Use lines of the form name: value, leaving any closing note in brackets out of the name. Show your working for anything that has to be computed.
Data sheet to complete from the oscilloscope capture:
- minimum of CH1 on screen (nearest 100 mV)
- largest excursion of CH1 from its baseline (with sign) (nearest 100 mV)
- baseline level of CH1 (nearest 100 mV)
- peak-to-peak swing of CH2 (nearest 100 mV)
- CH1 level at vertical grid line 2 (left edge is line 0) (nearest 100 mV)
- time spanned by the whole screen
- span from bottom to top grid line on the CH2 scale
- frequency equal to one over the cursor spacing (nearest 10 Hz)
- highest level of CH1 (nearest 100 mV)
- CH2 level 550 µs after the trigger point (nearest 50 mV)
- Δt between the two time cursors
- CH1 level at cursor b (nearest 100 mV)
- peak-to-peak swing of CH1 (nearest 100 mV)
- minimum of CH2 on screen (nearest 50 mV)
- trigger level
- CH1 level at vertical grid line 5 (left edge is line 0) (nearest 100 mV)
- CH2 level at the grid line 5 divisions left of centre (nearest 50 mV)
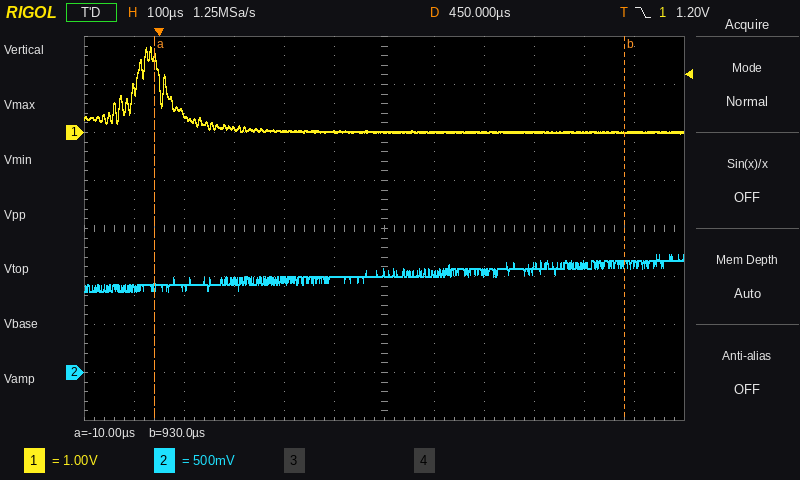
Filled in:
minimum of CH1 on screen: 0.0 V
largest excursion of CH1 from its baseline (with sign): 1.8 V − (0.0 V) = +1.8 V
baseline level of CH1: 0.0 V
peak-to-peak swing of CH2: 400 mV
CH1 level at vertical grid line 2 (left edge is line 0): 400 mV
time spanned by the whole screen: 1.2 ms
span from bottom to top grid line on the CH2 scale: 4 V
frequency equal to one over the cursor spacing: 1 / 940 µs ≈ 1.06 kHz
highest level of CH1: 1.8 V
CH2 level 550 µs after the trigger point: 1.05 V
Δt between the two time cursors: 930 µs − (-10 µs) = 940 µs
CH1 level at cursor b: 0.0 V
peak-to-peak swing of CH1: 1.8 V − (0.0 V) = 1.8 V
minimum of CH2 on screen: 850 mV
trigger level: 1.20 V
CH1 level at vertical grid line 5 (left edge is line 0): 0.0 V
CH2 level at the grid line 5 divisions left of centre: 900 mV
